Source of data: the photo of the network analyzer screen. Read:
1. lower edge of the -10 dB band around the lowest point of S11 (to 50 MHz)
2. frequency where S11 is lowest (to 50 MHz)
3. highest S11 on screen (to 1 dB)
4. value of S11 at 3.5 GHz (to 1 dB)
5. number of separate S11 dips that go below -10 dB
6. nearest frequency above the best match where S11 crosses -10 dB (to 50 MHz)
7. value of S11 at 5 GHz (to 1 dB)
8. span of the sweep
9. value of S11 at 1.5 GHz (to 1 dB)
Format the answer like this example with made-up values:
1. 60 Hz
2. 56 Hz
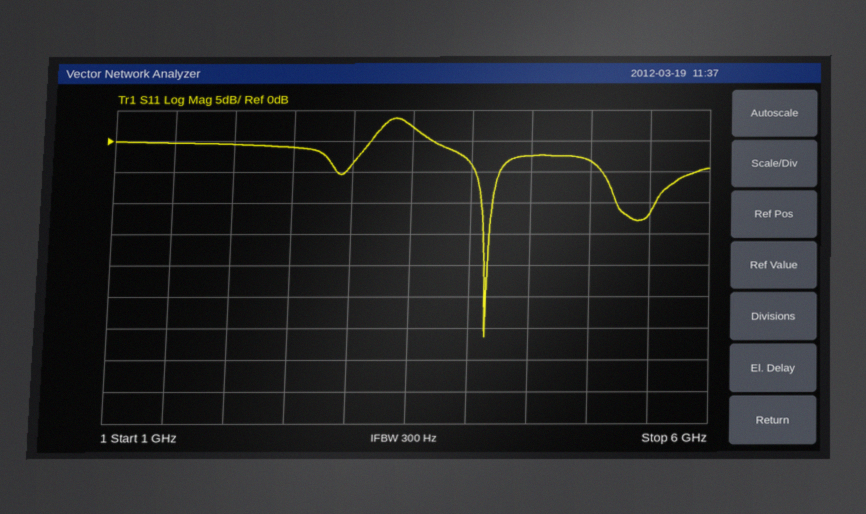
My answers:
1. 4.10 GHz
2. 4.15 GHz
3. 4 dB
4. 2 dB
5. 2
6. 4.20 GHz
7. -3 dB
8. 5 GHz
9. 0 dB
